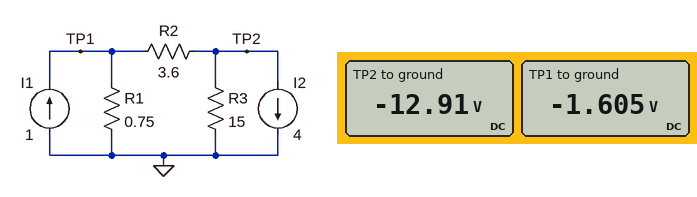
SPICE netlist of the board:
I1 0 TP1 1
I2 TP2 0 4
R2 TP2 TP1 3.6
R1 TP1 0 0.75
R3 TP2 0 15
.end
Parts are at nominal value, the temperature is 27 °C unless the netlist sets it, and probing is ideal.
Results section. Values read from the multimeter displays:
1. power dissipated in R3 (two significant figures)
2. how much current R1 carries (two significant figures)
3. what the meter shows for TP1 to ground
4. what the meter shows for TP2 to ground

11 W
2.1 A
-1.605 V
-12.91 V
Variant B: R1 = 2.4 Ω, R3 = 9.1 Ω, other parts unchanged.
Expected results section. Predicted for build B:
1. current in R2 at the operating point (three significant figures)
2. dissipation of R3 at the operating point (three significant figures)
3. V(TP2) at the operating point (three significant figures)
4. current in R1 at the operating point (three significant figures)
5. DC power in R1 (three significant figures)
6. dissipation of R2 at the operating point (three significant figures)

2.57 A
18.6 W
-13.0 V
1.57 A
5.91 W
23.8 W
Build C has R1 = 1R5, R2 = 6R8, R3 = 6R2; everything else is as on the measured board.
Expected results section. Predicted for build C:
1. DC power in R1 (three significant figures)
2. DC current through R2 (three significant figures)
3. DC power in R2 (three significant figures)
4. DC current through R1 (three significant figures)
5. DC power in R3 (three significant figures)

993 mW
1.81 A
22.4 W
814 mA
29.6 W
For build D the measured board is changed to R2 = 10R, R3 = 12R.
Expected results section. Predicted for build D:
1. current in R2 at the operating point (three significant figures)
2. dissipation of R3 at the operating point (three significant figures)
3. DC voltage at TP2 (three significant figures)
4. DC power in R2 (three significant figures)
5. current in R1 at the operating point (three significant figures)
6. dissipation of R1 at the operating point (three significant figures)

2.14 A
41.4 W
-22.3 V
45.9 W
1.14 A
980 mW
